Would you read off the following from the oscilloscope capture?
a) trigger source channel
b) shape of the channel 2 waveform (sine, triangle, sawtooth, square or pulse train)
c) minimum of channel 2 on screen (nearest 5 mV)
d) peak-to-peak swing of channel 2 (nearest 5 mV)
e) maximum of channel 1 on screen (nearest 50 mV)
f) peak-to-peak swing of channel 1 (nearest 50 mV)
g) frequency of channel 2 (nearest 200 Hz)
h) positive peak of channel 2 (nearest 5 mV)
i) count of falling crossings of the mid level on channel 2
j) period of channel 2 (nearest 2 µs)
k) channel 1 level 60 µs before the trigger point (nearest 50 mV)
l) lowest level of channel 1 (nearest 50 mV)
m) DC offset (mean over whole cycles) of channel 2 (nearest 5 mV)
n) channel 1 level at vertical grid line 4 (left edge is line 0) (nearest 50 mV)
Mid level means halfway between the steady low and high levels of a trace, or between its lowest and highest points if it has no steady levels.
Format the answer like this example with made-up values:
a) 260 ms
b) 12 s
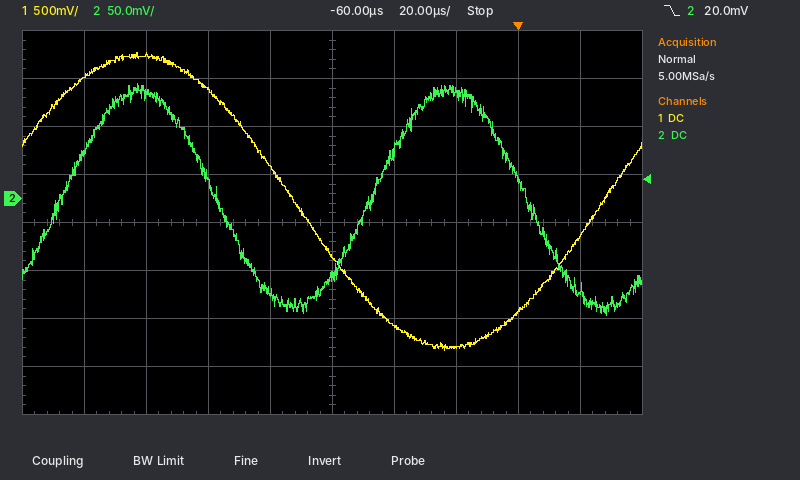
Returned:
a) channel 2
b) sine
c) -120 mV
d) 240 mV
e) 1.50 V
f) 3.10 V
g) 10.0 kHz
h) 120 mV
i) 2
j) 100 µs
k) -600 mV
l) -1.60 V
m) 0 mV
n) 350 mV
